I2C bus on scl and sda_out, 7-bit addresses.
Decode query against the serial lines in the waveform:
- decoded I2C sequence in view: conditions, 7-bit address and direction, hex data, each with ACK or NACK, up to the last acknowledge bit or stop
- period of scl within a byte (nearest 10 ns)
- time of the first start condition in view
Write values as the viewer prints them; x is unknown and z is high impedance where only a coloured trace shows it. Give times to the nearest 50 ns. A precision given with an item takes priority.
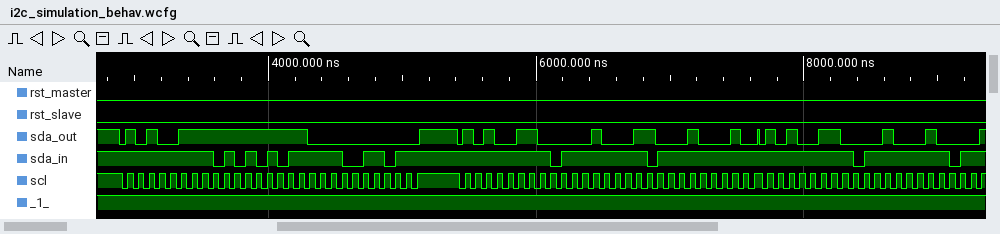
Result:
start, address 53 read NACK, FF ACK, 00 ACK, stop, start, address 53 write ACK, 11 NACK, 11 ACK, stop, start, address 53 write ACK, 22 ACK
80 ns
2900 ns
